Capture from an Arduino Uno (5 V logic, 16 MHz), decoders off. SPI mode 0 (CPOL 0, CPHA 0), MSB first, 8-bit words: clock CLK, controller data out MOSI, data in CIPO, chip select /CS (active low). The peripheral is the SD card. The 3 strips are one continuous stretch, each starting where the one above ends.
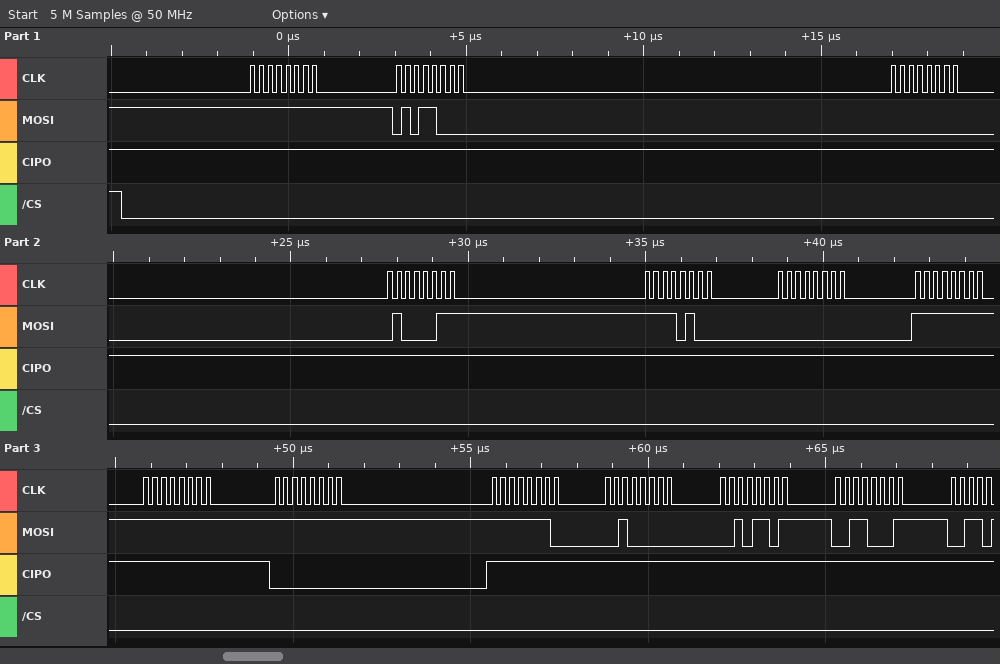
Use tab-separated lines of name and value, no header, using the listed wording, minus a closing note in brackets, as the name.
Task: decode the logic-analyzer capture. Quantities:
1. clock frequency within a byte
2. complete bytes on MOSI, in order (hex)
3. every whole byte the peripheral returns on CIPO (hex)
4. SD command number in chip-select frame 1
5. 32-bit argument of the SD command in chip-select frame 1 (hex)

clock frequency within a byte	4 MHz
complete bytes on MOSI, in order	FF 58 00 43 F4 00 FF FF FF FE 20 2D 31
every whole byte the peripheral returns on CIPO	FF FF FF FF FF FF FF FF 00 FF FF FF FF
SD command number in chip-select frame 1	CMD24
32-bit argument of the SD command in chip-select frame 1	0x0043F400
